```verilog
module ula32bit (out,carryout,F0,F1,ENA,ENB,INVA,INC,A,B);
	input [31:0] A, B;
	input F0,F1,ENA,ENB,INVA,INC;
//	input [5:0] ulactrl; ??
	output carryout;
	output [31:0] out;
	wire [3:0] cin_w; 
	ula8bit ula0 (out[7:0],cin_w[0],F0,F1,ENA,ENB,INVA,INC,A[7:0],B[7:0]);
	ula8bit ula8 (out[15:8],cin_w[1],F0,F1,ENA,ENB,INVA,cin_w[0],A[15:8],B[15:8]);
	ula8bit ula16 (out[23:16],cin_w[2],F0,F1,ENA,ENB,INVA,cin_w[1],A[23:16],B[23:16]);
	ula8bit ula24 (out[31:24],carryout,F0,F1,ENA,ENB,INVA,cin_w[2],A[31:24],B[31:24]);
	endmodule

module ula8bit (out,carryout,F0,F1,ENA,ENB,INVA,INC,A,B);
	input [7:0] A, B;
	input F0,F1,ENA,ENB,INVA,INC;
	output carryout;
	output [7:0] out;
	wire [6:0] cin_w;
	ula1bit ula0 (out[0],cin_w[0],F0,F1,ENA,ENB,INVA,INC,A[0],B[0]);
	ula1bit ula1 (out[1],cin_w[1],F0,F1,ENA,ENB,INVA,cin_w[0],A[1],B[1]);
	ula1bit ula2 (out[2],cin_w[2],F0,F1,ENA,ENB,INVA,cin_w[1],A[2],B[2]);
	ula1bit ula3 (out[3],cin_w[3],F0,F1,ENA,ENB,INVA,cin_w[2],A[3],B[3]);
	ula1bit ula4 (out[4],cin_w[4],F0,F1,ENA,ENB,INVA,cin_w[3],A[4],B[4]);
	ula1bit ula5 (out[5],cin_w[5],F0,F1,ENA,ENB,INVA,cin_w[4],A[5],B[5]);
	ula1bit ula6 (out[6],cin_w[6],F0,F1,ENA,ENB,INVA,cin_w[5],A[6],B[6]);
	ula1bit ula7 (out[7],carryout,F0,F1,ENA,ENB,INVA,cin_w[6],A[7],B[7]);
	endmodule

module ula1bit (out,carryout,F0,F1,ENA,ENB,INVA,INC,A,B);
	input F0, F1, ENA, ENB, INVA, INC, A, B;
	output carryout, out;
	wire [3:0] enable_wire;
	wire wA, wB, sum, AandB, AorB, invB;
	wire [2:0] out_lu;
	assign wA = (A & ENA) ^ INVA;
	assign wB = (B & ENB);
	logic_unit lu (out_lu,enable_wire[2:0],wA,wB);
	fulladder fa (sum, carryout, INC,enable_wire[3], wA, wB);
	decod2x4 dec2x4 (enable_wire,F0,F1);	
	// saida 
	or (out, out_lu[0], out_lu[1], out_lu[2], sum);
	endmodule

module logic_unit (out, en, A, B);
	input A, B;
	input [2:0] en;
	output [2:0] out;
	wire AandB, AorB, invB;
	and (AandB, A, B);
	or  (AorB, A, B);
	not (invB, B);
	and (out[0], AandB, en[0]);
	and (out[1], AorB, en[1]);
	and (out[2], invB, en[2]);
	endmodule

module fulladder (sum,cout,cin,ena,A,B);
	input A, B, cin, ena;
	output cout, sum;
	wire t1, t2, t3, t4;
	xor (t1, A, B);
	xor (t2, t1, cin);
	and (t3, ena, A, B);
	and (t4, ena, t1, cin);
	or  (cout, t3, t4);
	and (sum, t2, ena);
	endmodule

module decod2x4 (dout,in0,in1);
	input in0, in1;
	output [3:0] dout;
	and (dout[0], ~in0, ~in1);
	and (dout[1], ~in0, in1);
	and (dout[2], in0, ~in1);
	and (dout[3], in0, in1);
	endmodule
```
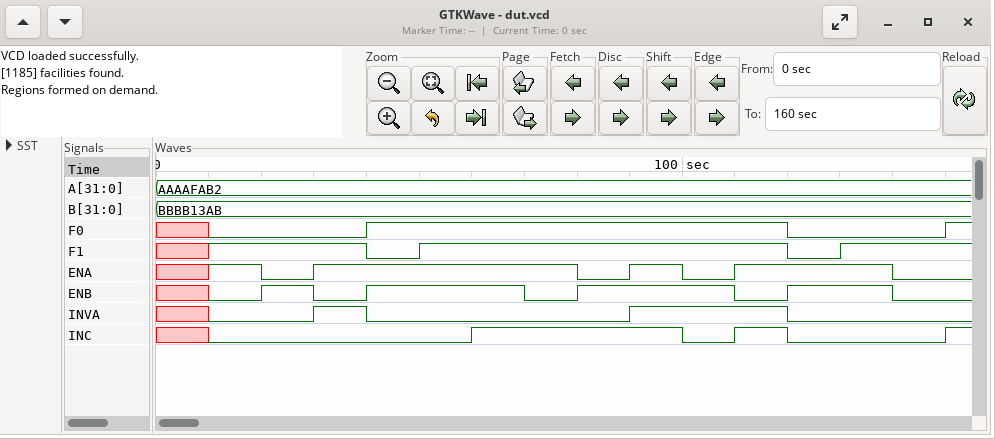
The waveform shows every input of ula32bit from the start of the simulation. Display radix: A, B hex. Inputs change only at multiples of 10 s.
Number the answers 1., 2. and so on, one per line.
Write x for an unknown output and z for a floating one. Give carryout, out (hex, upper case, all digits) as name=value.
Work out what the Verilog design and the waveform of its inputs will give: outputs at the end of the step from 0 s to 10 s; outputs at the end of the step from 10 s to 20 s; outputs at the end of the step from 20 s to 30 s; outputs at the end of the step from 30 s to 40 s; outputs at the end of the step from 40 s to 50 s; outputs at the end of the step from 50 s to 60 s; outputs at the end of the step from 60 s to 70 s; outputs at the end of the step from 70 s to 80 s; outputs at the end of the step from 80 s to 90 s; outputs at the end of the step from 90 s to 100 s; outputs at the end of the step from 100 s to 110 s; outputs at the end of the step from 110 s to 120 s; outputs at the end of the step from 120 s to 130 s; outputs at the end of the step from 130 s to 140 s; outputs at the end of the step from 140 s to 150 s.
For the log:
1. carryout=x, out=x
2. carryout=0, out=AAAAFAB2
3. carryout=0, out=BBBB13AB
4. carryout=0, out=5555054D
5. carryout=0, out=4444EC54
6. carryout=1, out=66660E5D
7. carryout=1, out=66660E5E
8. carryout=0, out=AAAAFAB3
9. carryout=0, out=BBBB13AC
10. carryout=1, out=111018F9
11. carryout=1, out=BBBB13AA
12. carryout=0, out=5555054E
13. carryout=0, out=AAAA12A2
14. carryout=0, out=BBBBFBBB
15. carryout=0, out=00000000
